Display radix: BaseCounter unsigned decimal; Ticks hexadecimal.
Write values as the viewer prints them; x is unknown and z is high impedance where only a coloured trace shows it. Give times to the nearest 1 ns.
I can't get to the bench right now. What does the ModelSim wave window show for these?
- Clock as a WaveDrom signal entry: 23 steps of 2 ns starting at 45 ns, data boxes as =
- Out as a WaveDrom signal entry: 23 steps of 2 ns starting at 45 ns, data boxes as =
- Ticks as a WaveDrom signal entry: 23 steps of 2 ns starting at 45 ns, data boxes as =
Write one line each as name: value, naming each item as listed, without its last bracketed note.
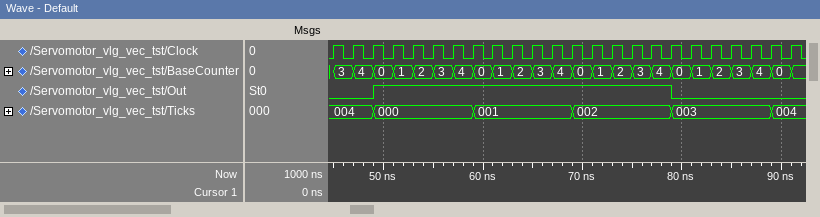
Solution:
Clock as a WaveDrom signal entry: 23 steps of 2 ns starting at 45 ns, data boxes as =: {name: 'Clock', wave: 'p......................'}
Out as a WaveDrom signal entry: 23 steps of 2 ns starting at 45 ns, data boxes as =: {name: 'Out', wave: '0.1..............0.....'}
Ticks as a WaveDrom signal entry: 23 steps of 2 ns starting at 45 ns, data boxes as =: {name: 'Ticks', wave: '=.=....=....=....=....=', data: '004 000 001 002 003 004'}
